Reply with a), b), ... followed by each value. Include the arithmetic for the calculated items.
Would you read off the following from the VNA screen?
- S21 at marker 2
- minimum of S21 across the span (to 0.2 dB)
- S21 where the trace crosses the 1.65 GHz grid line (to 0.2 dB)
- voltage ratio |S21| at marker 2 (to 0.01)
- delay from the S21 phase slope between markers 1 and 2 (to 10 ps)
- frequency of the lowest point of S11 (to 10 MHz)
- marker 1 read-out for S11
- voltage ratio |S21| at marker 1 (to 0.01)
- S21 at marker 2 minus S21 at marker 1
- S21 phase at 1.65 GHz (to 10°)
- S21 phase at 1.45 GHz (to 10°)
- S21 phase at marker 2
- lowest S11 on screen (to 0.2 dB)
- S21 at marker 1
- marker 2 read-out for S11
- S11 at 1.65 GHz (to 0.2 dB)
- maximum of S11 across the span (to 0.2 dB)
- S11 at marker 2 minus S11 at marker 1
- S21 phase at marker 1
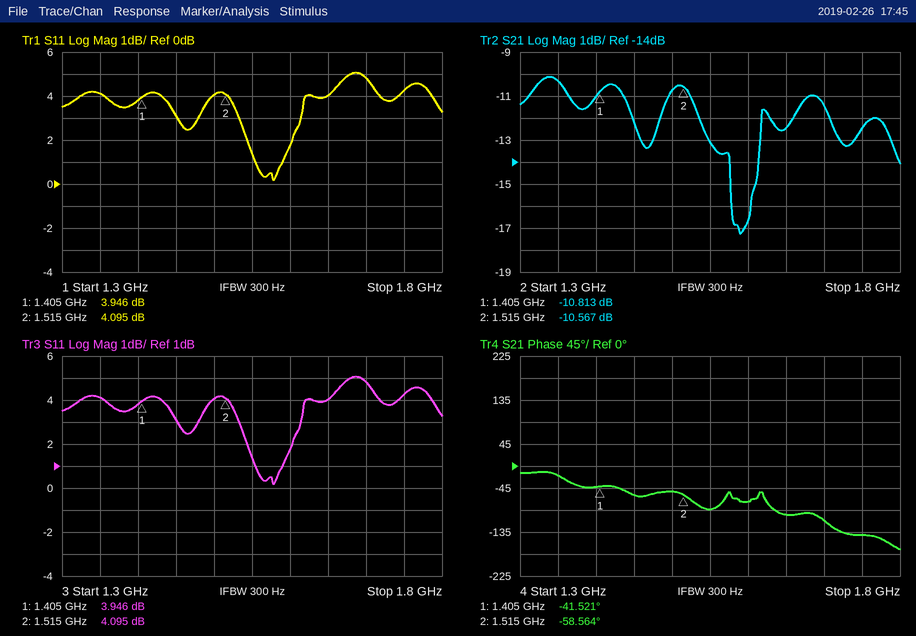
a) -10.567 dB
b) -17.2 dB
c) -12.4 dB
d) 10^(-10.567/20) ≈ 0.30
e) −(-58.564° − (-41.521°))/(360° × 110 MHz) ≈ 430 ps
f) 1.58 GHz
g) 3.946 dB
h) 10^(-10.813/20) ≈ 0.29
i) -10.567 − (-10.813) = 0.246 dB
j) -100°
k) -60°
l) -58.564°
m) 0.2 dB
n) -10.813 dB
o) 4.095 dB
p) 4.0 dB
q) 5.0 dB
r) 4.095 − (3.946) = 0.149 dB
s) -41.521°
